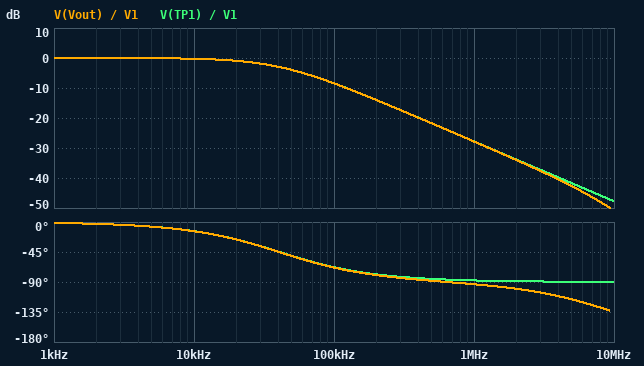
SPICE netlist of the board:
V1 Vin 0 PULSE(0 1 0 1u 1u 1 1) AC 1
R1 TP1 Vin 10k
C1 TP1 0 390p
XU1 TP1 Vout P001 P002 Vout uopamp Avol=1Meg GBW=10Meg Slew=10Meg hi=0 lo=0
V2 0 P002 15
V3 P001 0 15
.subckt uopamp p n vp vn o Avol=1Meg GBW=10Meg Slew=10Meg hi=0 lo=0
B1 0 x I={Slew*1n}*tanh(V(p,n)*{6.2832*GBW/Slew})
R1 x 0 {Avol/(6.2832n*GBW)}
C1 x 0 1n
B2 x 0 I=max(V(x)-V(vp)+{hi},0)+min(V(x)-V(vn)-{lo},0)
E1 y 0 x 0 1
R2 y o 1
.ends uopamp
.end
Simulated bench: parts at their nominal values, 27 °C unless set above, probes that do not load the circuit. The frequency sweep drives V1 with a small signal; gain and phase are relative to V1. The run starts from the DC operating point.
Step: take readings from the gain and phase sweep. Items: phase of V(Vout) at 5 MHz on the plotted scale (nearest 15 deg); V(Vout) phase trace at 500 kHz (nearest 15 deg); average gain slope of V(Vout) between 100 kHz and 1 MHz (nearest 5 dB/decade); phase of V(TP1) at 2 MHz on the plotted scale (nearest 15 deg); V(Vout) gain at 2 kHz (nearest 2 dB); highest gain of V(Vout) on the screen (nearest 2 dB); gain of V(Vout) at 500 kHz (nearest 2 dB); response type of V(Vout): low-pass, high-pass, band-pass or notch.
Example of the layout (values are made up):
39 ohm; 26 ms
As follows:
-120 deg; -90 deg; -20 dB/decade; -90 deg; 0 dB; 0 dB; -22 dB; low-pass
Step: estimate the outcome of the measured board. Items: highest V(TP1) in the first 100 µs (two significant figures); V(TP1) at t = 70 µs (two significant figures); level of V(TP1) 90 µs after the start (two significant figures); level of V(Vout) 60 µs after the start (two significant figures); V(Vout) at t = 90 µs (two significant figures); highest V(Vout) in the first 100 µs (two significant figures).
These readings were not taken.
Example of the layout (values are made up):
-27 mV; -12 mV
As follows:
1.0 V; 1.0 V; 1.0 V; 1.0 V; 1.0 V; 1.0 V
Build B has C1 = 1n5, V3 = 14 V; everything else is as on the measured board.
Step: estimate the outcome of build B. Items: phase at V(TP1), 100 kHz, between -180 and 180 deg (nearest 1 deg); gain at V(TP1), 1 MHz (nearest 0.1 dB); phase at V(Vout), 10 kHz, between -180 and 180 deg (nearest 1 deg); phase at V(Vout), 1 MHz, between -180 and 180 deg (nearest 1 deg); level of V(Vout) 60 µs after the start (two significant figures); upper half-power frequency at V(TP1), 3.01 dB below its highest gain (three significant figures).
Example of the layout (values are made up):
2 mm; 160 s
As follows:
-84 deg; -39.5 dB; -43 deg; -95 deg; 980 mV; 10.6 kHz
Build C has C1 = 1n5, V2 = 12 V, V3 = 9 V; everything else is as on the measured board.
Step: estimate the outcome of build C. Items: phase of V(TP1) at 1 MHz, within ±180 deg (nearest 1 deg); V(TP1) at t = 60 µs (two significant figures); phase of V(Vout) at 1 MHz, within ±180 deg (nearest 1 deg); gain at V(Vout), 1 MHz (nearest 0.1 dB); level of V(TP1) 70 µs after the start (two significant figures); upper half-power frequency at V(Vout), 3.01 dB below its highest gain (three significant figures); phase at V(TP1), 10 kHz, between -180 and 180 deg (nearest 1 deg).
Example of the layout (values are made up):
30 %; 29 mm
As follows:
-89 deg; 980 mV; -95 deg; -39.5 dB; 990 mV; 10.6 kHz; -43 deg
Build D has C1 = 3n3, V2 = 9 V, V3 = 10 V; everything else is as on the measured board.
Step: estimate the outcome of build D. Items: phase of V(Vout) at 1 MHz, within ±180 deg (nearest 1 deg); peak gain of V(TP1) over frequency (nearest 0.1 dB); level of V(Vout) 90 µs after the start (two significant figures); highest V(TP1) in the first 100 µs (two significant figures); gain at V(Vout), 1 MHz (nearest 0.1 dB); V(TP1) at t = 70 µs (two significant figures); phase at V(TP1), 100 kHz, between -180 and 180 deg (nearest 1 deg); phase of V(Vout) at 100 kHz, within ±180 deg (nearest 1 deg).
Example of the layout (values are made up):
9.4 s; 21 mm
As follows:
-95 deg; 0 dB; 930 mV; 950 mV; -46.4 dB; 880 mV; -87 deg; -88 deg
